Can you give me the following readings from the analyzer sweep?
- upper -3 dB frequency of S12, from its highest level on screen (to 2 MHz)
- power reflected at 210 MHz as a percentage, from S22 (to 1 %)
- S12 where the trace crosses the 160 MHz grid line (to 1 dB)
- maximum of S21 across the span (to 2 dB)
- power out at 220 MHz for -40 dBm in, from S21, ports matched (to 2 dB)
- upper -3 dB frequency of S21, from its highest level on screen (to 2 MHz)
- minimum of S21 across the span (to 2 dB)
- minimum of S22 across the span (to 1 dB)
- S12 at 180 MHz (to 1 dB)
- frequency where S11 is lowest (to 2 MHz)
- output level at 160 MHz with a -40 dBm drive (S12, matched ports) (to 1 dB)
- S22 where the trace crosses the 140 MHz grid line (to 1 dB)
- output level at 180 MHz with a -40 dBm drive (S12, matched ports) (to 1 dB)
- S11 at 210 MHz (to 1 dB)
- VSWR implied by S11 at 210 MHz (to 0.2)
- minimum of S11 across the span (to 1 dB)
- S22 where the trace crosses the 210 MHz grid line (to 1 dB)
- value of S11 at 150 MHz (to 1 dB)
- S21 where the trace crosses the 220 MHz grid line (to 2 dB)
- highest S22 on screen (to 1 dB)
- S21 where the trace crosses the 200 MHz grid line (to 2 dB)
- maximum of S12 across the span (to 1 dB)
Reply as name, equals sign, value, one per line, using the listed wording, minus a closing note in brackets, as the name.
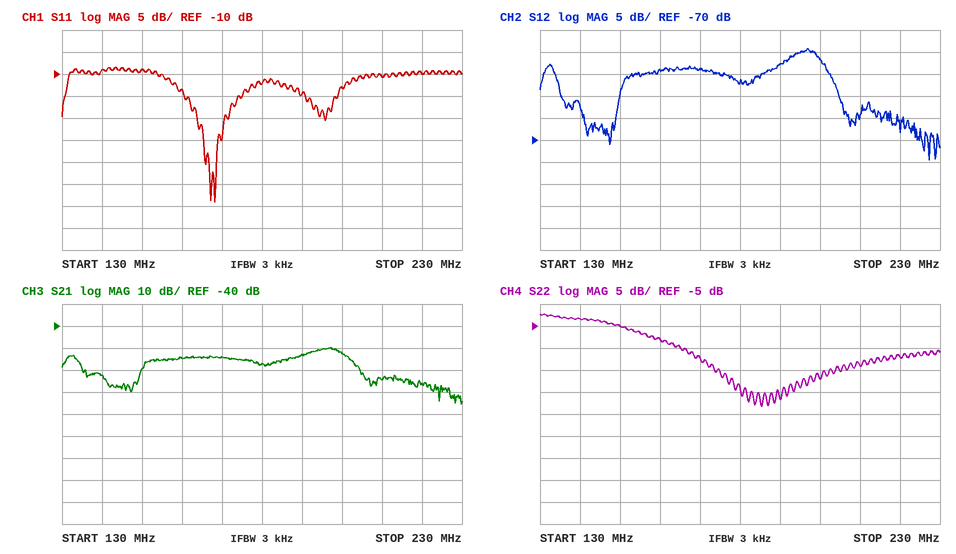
upper -3 dB frequency of S12, from its highest level on screen = 200 MHz
power reflected at 210 MHz as a percentage, from S22 = 4 %
S12 where the trace crosses the 160 MHz grid line = -54 dB
maximum of S21 across the span = -50 dB
power out at 220 MHz for -40 dBm in, from S21, ports matched = -106 dBm
upper -3 dB frequency of S21, from its highest level on screen = 200 MHz
minimum of S21 across the span = -76 dB
minimum of S22 across the span = -23 dB
S12 at 180 MHz = -57 dB
frequency where S11 is lowest = 168 MHz
output level at 160 MHz with a -40 dBm drive (S12, matched ports) = -94 dBm
S22 where the trace crosses the 140 MHz grid line = -3 dB
output level at 180 MHz with a -40 dBm drive (S12, matched ports) = -97 dBm
S11 at 210 MHz = -11 dB
VSWR implied by S11 at 210 MHz = 1.8
minimum of S11 across the span = -39 dB
S22 where the trace crosses the 210 MHz grid line = -14 dB
value of S11 at 150 MHz = -9 dB
S21 where the trace crosses the 220 MHz grid line = -66 dB
highest S22 on screen = -2 dB
S21 where the trace crosses the 200 MHz grid line = -52 dB
maximum of S12 across the span = -49 dB
